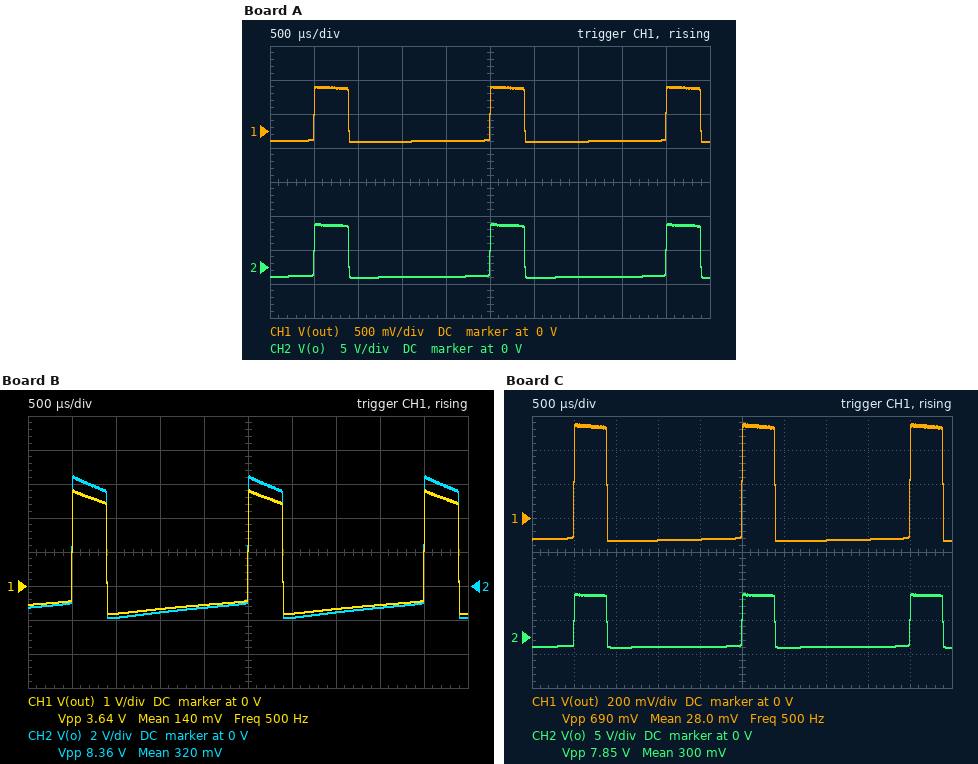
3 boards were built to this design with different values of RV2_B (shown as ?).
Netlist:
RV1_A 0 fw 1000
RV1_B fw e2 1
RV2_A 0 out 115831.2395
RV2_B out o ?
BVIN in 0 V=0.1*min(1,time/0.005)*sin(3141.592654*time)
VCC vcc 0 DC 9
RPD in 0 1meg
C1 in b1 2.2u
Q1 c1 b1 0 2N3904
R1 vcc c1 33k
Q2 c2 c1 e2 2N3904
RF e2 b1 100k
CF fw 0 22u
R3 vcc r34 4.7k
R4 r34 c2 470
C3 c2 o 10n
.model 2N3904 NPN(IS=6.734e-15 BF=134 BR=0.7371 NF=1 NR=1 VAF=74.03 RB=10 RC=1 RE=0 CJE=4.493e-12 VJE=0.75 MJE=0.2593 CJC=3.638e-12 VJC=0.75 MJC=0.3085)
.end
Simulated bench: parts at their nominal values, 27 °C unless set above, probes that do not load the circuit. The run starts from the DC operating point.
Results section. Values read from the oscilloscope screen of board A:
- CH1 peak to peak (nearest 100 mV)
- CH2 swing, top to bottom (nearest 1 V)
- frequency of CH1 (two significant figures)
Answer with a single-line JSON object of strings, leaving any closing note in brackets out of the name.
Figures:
{"CH1 peak to peak": "800 mV", "CH2 swing, top to bottom": "8 V", "frequency of CH1": "500 Hz"}
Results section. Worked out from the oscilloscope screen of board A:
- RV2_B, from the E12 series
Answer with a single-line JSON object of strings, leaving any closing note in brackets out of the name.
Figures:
{"RV2_B, from the E12 series": "1 MΩ"}
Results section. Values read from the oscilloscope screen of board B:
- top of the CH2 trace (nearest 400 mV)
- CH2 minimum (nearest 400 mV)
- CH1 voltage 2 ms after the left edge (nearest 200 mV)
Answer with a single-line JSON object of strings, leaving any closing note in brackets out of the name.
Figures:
{"top of the CH2 trace": "6.4 V", "CH2 minimum": "-2.0 V", "CH1 voltage 2 ms after the left edge": "-600 mV"}
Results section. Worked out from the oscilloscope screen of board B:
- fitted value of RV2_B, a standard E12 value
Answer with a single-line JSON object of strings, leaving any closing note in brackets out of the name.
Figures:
{"fitted value of RV2_B, a standard E12 value": "150 kΩ"}
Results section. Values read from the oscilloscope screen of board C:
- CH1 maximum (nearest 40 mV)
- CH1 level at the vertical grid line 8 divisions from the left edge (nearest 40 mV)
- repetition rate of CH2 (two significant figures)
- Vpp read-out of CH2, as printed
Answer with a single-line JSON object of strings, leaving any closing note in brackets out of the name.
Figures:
{"CH1 maximum": "560 mV", "CH1 level at the vertical grid line 8 divisions from the left edge": "-120 mV", "repetition rate of CH2": "500 Hz", "Vpp read-out of CH2, as printed": "7.85 V"}
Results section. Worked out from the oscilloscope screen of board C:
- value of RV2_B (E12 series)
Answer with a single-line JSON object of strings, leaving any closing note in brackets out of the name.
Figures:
{"value of RV2_B": "1.2 MΩ"}
